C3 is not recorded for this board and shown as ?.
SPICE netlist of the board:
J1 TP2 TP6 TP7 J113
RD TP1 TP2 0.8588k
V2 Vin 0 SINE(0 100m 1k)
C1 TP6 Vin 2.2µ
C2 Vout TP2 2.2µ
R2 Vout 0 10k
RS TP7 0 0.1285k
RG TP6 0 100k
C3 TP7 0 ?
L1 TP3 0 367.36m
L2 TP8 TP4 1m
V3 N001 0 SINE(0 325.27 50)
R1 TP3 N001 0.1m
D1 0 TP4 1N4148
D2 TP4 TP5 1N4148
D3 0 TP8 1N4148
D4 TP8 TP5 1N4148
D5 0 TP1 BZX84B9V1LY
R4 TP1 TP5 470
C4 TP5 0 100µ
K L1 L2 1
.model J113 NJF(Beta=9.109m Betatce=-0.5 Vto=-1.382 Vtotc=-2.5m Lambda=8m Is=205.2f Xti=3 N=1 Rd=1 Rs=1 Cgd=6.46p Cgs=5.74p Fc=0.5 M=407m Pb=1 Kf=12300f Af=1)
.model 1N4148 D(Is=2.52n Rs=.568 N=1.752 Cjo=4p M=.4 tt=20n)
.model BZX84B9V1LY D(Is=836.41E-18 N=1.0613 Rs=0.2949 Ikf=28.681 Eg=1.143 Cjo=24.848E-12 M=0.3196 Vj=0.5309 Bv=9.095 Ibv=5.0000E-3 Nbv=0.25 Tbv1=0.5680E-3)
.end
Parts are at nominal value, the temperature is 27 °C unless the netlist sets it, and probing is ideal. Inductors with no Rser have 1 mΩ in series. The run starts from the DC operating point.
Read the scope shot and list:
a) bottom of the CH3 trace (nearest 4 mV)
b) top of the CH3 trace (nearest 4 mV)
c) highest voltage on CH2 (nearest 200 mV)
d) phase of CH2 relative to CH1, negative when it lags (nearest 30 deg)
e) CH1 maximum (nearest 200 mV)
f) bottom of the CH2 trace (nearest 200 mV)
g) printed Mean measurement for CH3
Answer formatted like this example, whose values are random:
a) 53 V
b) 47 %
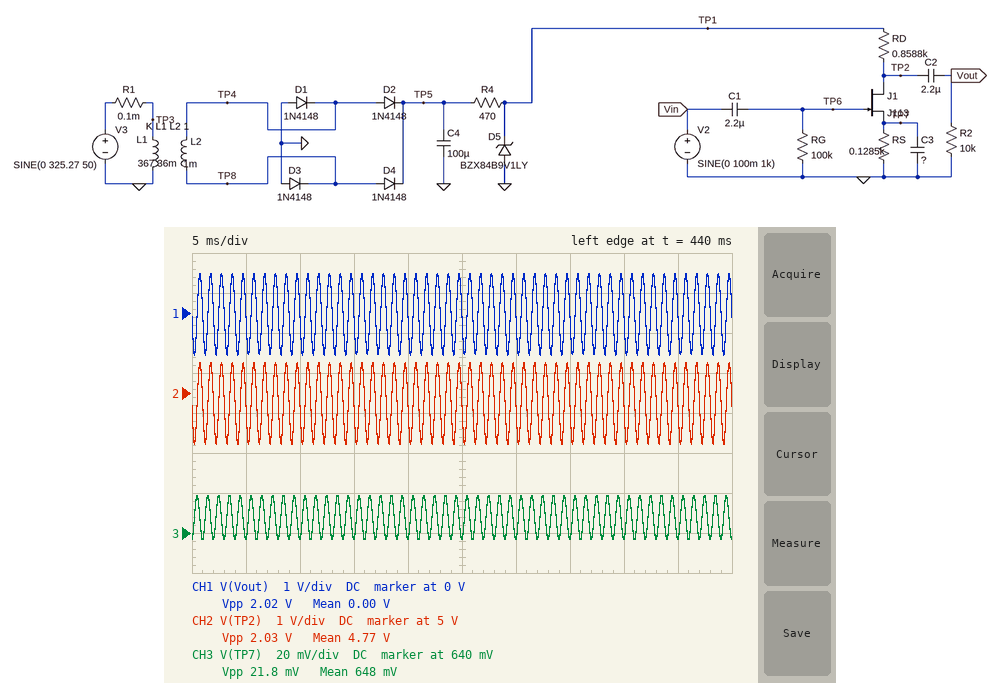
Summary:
a) 636 mV
b) 660 mV
c) 5.8 V
d) 0 deg
e) 1.0 V
f) 3.8 V
g) 648 mV
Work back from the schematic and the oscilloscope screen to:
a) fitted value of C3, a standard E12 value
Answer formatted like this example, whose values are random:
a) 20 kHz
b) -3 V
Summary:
a) 18 µF
